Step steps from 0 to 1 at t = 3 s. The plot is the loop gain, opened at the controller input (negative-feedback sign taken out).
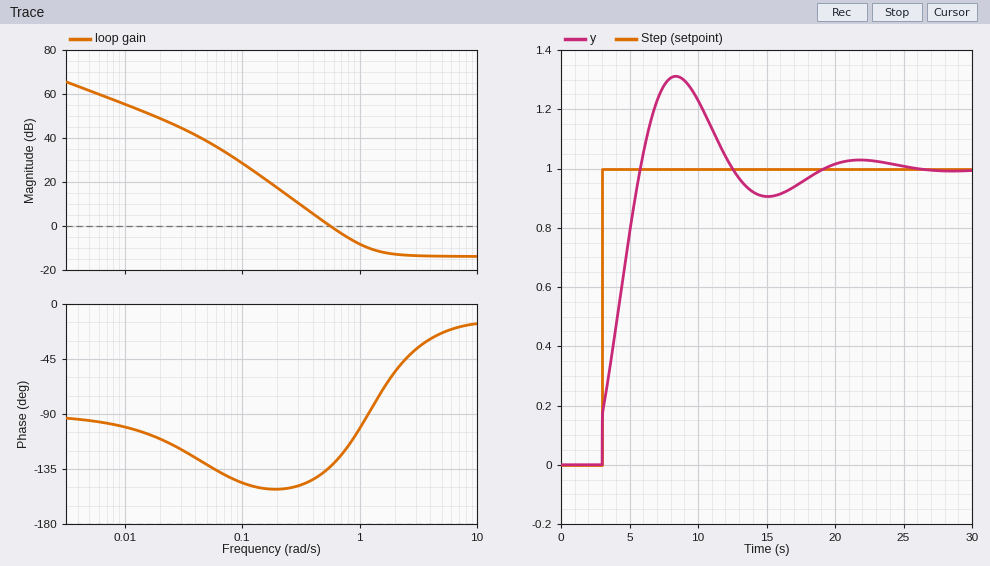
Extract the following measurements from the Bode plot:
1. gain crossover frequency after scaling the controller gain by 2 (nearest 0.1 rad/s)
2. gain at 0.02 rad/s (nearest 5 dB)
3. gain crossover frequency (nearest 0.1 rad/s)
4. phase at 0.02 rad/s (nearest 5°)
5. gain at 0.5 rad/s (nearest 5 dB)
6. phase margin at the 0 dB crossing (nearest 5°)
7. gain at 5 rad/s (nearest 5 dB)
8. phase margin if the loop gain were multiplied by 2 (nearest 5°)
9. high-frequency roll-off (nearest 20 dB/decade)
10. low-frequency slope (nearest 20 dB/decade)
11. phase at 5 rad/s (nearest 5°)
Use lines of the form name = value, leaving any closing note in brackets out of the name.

gain crossover frequency after scaling the controller gain by 2 = 0.8 rad/s
gain at 0.02 rad/s = 50 dB
gain crossover frequency = 0.6 rad/s
phase at 0.02 rad/s = -110°
gain at 0.5 rad/s = 0 dB
phase margin at the 0 dB crossing = 45°
gain at 5 rad/s = -15 dB
phase margin if the loop gain were multiplied by 2 = 65°
high-frequency roll-off = 0 dB/decade
low-frequency slope = -20 dB/decade
phase at 5 rad/s = -25°
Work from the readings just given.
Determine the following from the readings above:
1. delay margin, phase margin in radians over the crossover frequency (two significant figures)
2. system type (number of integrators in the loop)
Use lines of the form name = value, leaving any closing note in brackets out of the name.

delay margin, phase margin in radians over the crossover frequency = 1.3 s
system type = 1
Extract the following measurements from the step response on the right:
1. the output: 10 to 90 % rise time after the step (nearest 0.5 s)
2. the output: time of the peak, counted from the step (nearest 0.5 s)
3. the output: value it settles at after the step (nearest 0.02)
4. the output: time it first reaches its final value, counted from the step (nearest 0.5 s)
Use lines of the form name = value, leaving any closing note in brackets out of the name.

the output: 10 to 90 % rise time after the step = 2.5 s
the output: time of the peak, counted from the step = 5.5 s
the output: value it settles at after the step = 1.00
the output: time it first reaches its final value, counted from the step = 3.0 s
